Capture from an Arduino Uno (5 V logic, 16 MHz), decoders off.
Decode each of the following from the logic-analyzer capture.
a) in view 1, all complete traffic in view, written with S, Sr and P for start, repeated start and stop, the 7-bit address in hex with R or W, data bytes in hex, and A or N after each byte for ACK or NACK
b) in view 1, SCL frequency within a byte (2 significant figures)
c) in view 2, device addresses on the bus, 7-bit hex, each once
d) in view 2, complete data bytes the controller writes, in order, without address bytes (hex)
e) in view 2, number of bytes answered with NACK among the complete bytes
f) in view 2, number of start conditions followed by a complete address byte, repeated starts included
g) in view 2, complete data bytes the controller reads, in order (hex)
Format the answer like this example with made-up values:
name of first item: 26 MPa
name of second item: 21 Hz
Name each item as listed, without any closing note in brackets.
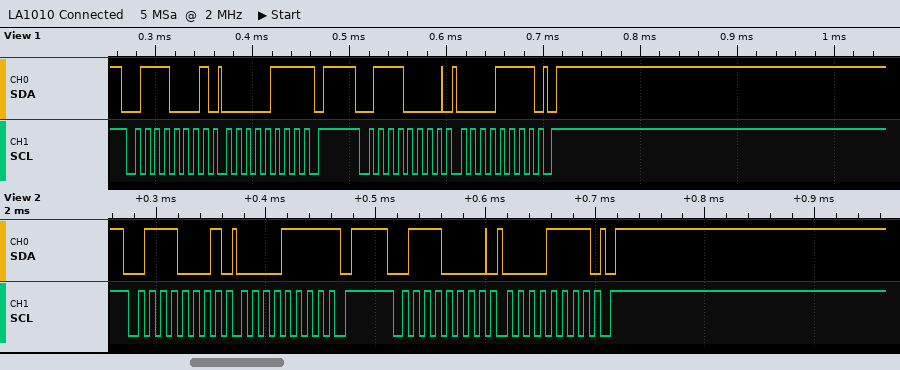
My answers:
in view 1, all complete traffic in view, written with S, Sr and P for start, repeated start and stop, the 7-bit address in hex with R or W, data bytes in hex, and A or N after each byte for ACK or NACK: S 38R A 07 N P S 38W A 0F A P
in view 1, SCL frequency within a byte: 100 kHz
in view 2, device addresses on the bus, 7-bit hex, each once: 0x38
in view 2, complete data bytes the controller writes, in order, without address bytes: 0F
in view 2, number of bytes answered with NACK among the complete bytes: 1
in view 2, number of start conditions followed by a complete address byte, repeated starts included: 2
in view 2, complete data bytes the controller reads, in order: 0F
